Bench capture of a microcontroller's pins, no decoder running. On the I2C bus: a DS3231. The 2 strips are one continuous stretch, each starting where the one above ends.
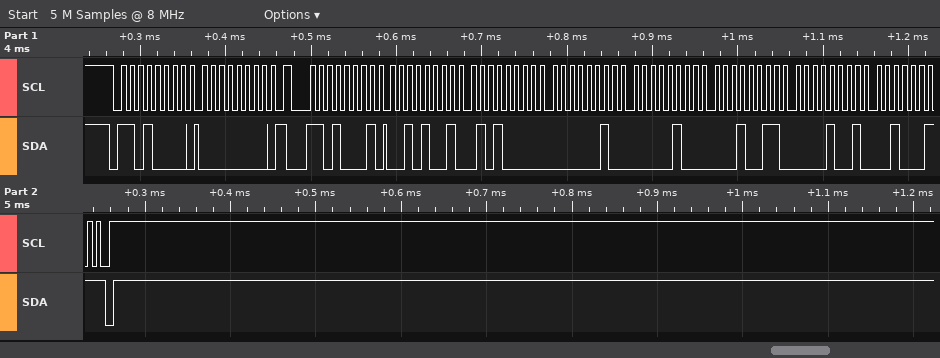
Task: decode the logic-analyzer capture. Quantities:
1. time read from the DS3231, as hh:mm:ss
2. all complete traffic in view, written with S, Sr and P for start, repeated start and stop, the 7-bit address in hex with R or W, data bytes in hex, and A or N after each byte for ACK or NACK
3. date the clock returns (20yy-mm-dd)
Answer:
02:50:29
S 68W A 00 A Sr 68R A 29 A 50 A 02 A 04 A 13 A 09 A 23 N P
2023-09-13
